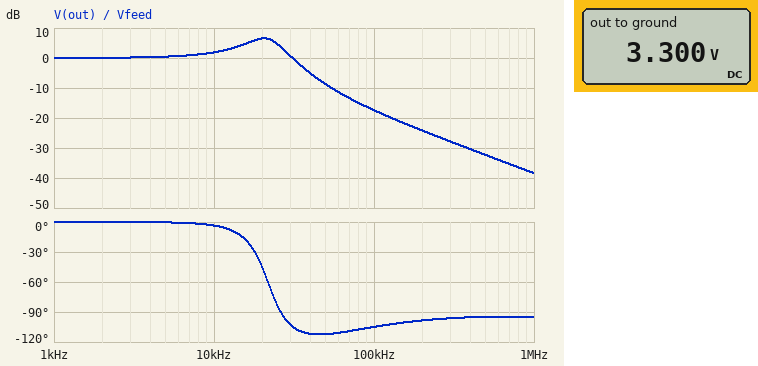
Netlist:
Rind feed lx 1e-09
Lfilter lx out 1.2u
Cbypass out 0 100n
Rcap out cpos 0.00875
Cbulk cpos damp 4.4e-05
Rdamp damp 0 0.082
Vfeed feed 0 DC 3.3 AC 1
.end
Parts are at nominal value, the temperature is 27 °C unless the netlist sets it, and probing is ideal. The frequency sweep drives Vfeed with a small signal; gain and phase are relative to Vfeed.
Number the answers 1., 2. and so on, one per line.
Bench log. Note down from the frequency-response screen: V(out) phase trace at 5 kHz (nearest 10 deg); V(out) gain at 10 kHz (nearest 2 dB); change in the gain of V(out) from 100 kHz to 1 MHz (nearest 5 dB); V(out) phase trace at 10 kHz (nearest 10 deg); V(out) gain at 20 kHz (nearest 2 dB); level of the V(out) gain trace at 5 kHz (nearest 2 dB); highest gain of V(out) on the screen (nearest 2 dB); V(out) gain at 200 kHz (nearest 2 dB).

1. 0 deg
2. 2 dB
3. -20 dB
4. 0 deg
5. 6 dB
6. 0 dB
7. 6 dB
8. -24 dB
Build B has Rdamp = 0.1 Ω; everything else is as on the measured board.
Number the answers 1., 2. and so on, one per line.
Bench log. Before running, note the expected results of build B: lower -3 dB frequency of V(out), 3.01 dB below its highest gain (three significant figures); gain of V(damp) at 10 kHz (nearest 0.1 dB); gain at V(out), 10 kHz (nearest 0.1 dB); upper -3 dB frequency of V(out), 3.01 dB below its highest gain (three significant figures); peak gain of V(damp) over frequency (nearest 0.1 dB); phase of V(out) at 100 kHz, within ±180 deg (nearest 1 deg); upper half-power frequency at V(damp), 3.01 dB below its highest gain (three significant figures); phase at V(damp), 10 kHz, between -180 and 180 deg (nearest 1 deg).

1. 11.6 kHz
2. -9.7 dB
3. 1.8 dB
4. 27.1 kHz
5. -0.7 dB
6. -100 deg
7. 30.2 kHz
8. 69 deg
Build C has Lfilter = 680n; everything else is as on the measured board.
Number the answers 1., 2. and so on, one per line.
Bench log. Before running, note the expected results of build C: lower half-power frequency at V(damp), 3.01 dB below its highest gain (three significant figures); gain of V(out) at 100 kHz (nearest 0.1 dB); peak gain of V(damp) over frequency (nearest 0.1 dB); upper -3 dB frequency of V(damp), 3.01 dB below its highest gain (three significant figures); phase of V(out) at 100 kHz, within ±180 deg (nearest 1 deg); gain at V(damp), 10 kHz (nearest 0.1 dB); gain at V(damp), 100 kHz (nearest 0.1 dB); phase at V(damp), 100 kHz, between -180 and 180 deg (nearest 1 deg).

1. 20.4 kHz
2. -12.3 dB
3. -0.9 dB
4. 41.5 kHz
5. -99 deg
6. -12.1 dB
7. -13.8 dB
8. -77 deg
